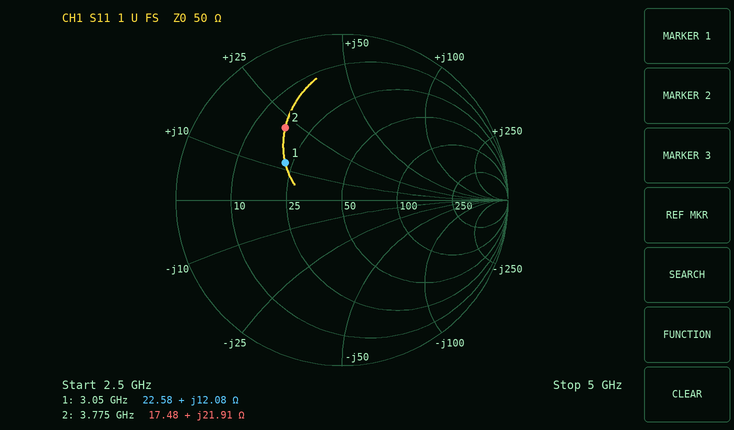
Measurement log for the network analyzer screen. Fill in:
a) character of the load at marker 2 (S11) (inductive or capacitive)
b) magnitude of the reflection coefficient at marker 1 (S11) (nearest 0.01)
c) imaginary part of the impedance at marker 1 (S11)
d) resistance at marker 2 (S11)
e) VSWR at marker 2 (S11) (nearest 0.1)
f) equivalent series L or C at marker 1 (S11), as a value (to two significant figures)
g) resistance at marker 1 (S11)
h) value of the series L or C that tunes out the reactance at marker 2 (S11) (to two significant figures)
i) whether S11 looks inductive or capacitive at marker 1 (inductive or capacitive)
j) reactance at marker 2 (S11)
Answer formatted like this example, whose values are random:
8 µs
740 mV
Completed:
inductive
0.41
+12.08 Ω
17.48 Ω
3.5
630 pH
22.58 Ω
1.9 pF
inductive
+21.91 Ω
